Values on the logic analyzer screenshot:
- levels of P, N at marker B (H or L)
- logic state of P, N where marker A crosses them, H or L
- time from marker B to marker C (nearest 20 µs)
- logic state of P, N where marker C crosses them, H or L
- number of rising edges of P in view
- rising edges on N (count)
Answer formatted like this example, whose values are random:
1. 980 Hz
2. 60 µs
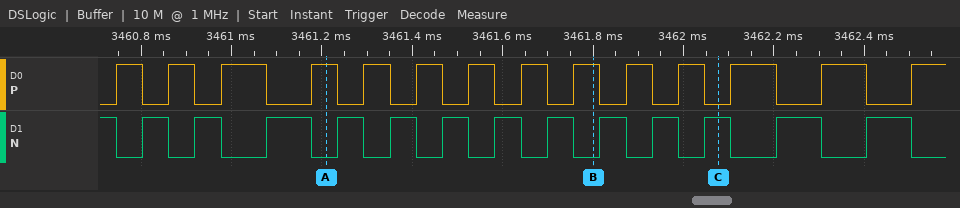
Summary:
1. P=H, N=L
2. P=H, N=L
3. 280 µs
4. P=L, N=H
5. 14
6. 13
